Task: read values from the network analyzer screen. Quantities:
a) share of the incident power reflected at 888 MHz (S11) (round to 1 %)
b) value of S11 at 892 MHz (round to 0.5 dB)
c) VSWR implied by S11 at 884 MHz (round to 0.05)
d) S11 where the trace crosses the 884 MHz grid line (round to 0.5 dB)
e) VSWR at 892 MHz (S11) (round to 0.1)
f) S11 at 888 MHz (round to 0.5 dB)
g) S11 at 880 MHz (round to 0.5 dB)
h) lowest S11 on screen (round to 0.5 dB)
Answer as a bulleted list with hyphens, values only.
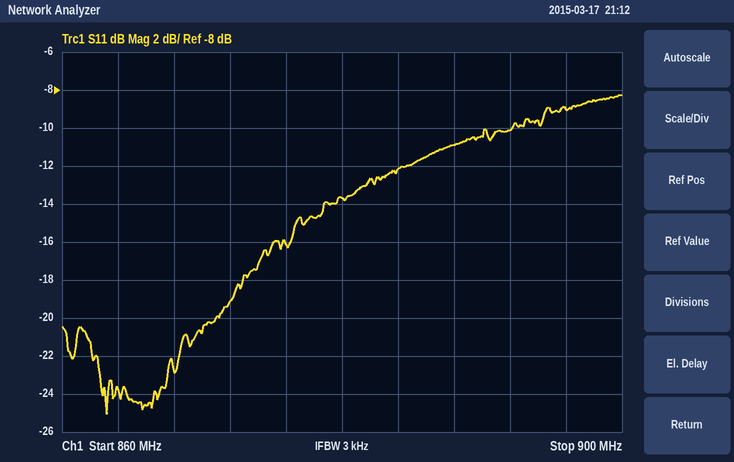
- 8 %
- -10.0 dB
- 1.65
- -12.0 dB
- 1.9
- -11.0 dB
- -13.5 dB
- -25.0 dB
